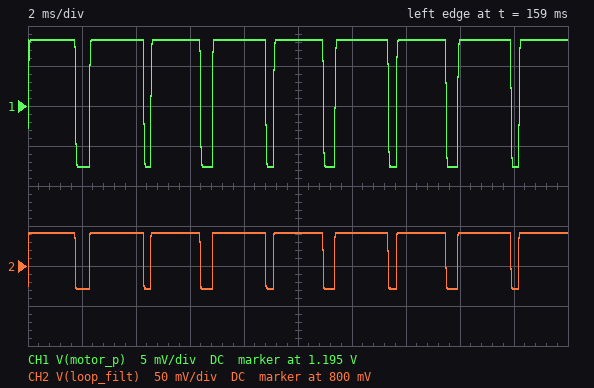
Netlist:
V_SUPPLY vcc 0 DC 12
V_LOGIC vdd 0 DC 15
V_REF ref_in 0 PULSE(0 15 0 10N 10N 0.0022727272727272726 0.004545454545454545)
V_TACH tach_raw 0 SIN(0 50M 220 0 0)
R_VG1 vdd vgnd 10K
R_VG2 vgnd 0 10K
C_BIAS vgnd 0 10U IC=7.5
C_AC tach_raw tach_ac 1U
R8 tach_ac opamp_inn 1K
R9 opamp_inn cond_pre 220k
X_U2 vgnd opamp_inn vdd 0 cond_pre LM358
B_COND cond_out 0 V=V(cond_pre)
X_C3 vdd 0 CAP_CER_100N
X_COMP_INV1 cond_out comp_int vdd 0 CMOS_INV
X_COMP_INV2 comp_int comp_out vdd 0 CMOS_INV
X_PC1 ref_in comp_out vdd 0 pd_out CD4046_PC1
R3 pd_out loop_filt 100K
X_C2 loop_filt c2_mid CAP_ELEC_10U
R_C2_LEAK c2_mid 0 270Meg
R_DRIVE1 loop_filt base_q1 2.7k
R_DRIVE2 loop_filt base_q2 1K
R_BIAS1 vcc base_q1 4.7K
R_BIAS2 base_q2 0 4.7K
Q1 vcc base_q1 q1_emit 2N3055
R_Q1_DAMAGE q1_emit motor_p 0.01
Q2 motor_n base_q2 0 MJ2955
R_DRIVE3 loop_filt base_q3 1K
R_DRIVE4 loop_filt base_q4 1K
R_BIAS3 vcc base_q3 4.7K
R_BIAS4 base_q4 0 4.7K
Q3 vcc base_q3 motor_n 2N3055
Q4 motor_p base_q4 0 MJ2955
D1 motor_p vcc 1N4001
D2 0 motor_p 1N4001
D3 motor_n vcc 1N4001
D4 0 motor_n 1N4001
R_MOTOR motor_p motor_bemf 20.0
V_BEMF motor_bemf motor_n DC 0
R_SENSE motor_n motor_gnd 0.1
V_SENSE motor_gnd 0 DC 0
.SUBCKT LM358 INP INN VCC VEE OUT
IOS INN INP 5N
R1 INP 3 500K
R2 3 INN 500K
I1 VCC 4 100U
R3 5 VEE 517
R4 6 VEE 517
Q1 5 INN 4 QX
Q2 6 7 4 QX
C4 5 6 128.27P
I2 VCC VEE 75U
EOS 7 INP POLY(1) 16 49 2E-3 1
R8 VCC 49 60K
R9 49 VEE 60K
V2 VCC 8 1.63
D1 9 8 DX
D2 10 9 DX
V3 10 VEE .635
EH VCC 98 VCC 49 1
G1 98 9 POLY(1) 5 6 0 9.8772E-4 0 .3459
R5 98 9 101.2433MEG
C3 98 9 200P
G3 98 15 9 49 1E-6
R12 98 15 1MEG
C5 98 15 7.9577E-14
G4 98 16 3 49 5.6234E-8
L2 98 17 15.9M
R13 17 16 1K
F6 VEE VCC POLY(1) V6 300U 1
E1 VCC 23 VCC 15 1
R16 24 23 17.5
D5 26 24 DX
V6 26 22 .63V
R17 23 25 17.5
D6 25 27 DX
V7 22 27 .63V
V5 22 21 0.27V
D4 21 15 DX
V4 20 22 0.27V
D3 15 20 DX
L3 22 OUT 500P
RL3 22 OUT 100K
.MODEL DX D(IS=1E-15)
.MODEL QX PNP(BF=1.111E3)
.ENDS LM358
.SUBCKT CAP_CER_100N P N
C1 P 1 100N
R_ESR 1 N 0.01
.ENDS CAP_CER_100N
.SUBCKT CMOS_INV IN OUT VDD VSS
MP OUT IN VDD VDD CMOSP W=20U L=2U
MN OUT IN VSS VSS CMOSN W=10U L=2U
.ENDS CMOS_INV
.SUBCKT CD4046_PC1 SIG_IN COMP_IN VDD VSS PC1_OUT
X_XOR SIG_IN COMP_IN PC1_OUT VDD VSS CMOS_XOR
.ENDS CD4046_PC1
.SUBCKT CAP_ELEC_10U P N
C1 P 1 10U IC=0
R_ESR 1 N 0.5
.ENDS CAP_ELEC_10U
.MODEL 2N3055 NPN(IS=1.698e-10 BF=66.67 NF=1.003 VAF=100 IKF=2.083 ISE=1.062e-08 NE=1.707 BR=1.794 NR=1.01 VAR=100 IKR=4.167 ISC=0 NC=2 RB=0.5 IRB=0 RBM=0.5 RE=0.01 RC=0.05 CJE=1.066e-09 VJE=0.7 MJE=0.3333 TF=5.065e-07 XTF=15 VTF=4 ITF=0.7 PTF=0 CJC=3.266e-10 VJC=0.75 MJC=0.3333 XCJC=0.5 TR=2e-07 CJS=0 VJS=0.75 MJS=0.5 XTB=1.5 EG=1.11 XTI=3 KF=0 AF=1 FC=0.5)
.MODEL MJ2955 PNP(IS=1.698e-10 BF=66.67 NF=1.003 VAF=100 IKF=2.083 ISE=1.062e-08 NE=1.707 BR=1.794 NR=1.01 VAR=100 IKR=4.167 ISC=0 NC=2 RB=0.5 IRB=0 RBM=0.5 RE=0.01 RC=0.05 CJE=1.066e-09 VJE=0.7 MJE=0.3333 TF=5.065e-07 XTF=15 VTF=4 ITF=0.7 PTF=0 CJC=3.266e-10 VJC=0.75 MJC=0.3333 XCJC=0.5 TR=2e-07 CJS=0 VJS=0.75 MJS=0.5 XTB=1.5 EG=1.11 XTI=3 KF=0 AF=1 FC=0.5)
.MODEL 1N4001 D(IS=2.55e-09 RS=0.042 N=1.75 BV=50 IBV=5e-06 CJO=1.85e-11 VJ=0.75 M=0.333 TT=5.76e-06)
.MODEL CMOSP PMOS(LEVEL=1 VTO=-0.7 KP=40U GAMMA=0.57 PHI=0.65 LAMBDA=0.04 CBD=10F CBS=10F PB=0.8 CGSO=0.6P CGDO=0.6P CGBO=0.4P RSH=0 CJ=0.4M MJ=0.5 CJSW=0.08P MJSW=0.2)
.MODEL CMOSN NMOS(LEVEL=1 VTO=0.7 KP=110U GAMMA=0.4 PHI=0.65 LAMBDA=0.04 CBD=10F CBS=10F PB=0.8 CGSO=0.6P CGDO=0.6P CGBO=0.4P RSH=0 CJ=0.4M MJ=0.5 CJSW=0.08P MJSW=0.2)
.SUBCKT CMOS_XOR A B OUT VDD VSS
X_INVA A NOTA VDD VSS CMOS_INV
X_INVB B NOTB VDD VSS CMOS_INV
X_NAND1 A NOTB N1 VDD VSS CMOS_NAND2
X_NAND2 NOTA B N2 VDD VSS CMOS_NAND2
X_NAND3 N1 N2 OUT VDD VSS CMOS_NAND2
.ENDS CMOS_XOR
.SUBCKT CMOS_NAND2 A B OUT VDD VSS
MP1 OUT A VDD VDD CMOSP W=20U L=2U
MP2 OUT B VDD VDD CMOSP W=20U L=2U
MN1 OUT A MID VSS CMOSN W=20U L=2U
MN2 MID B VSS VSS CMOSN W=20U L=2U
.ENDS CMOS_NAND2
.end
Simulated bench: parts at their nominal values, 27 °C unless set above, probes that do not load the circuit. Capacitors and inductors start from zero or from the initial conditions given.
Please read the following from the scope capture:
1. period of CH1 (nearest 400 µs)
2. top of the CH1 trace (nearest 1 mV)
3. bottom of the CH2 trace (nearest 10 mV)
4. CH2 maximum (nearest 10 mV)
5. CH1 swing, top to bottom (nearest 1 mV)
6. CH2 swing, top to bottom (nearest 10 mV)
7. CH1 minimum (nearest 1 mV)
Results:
2.4 ms
1.203 V
770 mV
840 mV
16 mV
70 mV
1.187 V
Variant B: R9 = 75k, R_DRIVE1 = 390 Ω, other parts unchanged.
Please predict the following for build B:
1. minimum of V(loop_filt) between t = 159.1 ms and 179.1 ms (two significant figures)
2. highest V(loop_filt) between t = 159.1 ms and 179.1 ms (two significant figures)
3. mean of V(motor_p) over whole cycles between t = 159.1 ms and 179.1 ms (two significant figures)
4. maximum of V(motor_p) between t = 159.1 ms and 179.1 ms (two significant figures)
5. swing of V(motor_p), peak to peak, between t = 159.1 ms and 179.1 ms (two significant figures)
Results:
1.0 V
1.1 V
890 mV
900 mV
41 mV
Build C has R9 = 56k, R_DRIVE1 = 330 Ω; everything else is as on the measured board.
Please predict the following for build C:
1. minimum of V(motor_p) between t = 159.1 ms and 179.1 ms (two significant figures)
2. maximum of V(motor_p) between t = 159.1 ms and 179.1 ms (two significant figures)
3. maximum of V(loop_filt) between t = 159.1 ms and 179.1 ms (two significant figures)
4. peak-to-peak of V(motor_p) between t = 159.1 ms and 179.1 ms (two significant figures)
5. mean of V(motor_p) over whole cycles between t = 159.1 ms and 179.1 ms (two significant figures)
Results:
840 mV
880 mV
1.1 V
42 mV
870 mV
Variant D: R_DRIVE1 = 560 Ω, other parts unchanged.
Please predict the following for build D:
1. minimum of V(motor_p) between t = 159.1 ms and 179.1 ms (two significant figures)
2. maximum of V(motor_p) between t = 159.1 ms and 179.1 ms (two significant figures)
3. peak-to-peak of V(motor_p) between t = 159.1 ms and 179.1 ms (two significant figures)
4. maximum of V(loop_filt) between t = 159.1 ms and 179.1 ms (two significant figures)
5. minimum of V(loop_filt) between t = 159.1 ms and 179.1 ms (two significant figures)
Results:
900 mV
940 mV
37 mV
1.0 V
970 mV
